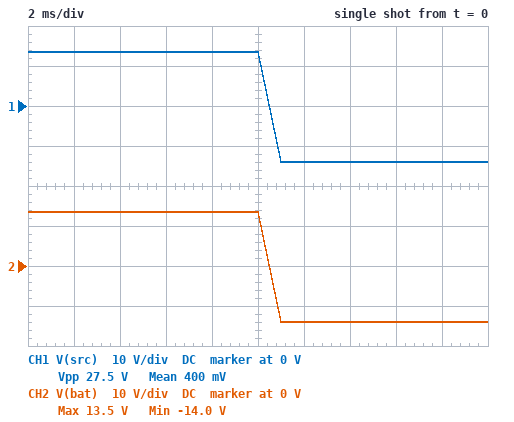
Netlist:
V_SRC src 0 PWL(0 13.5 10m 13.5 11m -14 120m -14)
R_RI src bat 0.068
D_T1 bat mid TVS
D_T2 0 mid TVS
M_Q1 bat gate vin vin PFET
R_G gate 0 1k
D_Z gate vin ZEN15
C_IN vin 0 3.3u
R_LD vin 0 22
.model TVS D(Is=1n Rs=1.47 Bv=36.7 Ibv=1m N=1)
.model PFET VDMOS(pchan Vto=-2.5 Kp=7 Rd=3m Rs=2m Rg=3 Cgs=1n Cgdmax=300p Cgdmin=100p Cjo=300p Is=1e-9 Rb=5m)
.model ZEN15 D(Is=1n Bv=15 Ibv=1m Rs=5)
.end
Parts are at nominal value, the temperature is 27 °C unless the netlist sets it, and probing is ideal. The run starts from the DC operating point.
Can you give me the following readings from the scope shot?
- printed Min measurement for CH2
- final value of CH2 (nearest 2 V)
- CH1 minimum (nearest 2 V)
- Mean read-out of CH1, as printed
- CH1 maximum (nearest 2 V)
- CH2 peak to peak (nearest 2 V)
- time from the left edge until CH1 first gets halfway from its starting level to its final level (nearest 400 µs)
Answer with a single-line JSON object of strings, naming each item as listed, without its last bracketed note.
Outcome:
{"printed Min measurement for CH2": "-14.0 V", "final value of CH2": "-14 V", "CH1 minimum": "-14 V", "Mean read-out of CH1, as printed": "400 mV", "CH1 maximum": "14 V", "CH2 peak to peak": "28 V", "time from the left edge until CH1 first gets halfway from its starting level to its final level": "10.4 ms"}
